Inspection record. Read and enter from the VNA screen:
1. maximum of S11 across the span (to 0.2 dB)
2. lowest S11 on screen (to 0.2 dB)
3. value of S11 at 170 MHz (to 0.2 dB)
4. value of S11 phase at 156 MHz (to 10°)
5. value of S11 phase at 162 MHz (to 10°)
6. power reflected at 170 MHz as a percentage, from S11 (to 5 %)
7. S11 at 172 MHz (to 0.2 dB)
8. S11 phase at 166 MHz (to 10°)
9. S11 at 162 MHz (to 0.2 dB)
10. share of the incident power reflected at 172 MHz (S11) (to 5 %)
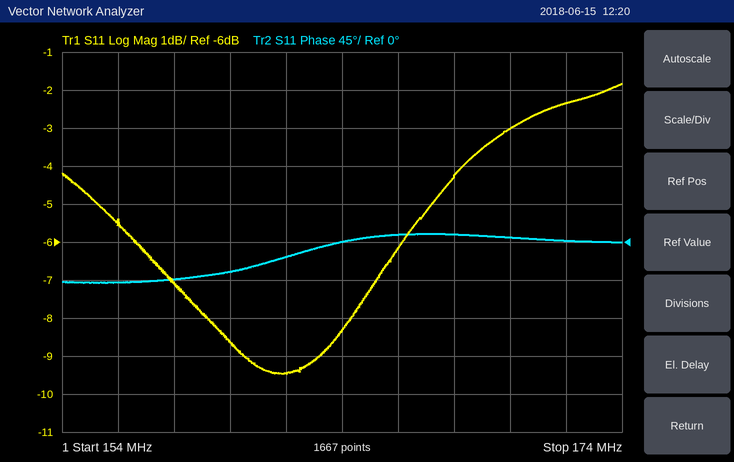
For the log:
-1.8 dB
-9.4 dB
-3.0 dB
-50°
-20°
50 %
-2.4 dB
10°
-9.4 dB
60 %
